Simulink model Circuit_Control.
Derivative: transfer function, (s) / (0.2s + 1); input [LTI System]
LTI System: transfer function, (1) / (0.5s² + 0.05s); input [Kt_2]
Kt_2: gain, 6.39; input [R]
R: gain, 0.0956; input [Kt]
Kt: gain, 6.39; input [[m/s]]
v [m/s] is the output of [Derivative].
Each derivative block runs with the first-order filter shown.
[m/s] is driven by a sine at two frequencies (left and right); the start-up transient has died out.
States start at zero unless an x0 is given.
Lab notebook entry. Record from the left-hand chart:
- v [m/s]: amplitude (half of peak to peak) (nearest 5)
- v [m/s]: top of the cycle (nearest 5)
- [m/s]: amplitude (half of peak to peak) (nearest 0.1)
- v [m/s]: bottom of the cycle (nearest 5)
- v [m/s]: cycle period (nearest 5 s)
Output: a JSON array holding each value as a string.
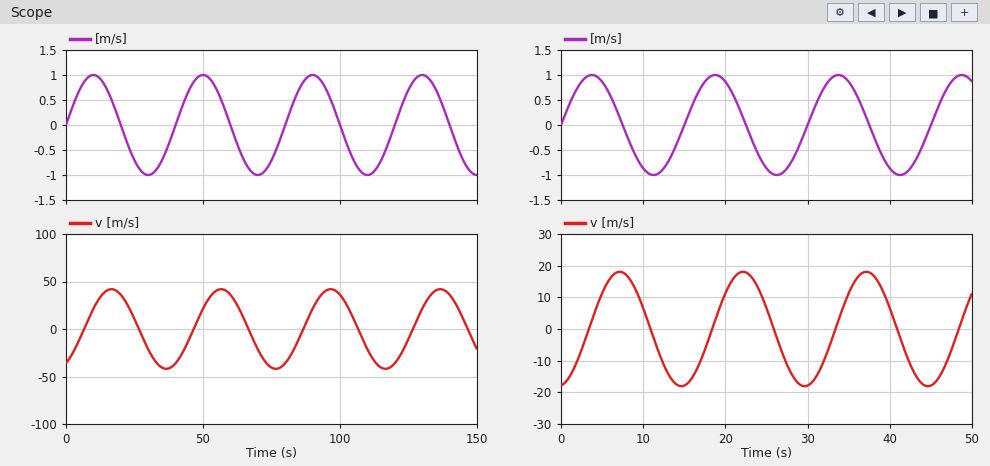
["40", "40", "1.0", "-40", "40 s"]
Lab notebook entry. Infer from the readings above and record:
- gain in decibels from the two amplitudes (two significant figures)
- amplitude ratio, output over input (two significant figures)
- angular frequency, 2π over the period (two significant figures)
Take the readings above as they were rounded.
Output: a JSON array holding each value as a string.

["32 dB", "40", "0.16 rad/s"]
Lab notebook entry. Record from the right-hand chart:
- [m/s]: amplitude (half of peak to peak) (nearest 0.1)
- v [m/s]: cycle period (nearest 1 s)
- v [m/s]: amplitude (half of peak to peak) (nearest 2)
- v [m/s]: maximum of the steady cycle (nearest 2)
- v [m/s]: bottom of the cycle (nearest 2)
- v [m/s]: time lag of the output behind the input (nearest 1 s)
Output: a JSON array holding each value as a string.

["1.0", "15 s", "18", "18", "-18", "3 s"]
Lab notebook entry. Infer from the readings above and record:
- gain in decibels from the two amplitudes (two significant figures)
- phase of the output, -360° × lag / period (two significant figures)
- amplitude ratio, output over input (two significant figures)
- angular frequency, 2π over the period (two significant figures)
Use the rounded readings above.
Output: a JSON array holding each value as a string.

["25 dB", "-72°", "18", "0.42 rad/s"]
